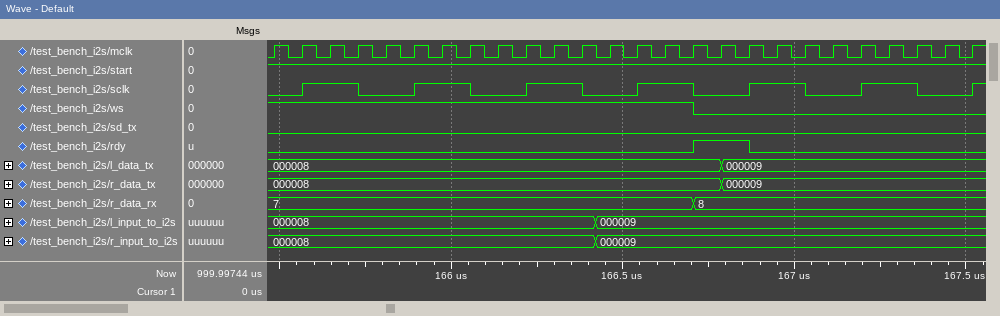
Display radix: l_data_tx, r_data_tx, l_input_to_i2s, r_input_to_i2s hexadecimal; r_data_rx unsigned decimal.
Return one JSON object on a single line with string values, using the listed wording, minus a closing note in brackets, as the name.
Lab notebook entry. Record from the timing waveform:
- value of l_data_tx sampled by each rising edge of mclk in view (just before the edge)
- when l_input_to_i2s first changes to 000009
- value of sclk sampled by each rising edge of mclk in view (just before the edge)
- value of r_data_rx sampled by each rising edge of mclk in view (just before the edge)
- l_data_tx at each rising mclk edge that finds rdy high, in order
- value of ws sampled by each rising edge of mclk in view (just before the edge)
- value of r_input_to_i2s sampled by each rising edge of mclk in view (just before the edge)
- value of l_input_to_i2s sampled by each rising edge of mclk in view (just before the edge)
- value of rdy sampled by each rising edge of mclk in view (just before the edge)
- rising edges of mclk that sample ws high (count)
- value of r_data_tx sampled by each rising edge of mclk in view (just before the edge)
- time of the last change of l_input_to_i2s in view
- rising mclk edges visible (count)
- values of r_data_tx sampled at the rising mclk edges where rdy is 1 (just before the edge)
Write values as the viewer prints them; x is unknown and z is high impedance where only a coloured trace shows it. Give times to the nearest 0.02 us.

{"value of l_data_tx sampled by each rising edge of mclk in view": "000008, 000008, 000008, 000008, 000008, 000008, 000008, 000008, 000008, 000008, 000008, 000008, 000008, 000008, 000008, 000008, 000008, 000009, 000009, 000009, 000009, 000009, 000009, 000009, 000009, 000009", "when l_input_to_i2s first changes to 000009": "166.42 us", "value of sclk sampled by each rising edge of mclk in view": "0 0 1 1 0 0 1 1 0 0 1 1 0 0 1 1 0 0 1 1 0 0 1 1 0 0", "value of r_data_rx sampled by each rising edge of mclk in view": "7, 7, 7, 7, 7, 7, 7, 7, 7, 7, 7, 7, 7, 7, 7, 7, 8, 8, 8, 8, 8, 8, 8, 8, 8, 8", "l_data_tx at each rising mclk edge that finds rdy high, in order": "000008, 000009", "value of ws sampled by each rising edge of mclk in view": "1 1 1 1 1 1 1 1 1 1 1 1 1 1 1 1 0 0 0 0 0 0 0 0 0 0", "value of r_input_to_i2s sampled by each rising edge of mclk in view": "000008, 000008, 000008, 000008, 000008, 000008, 000008, 000008, 000008, 000008, 000008, 000008, 000009, 000009, 000009, 000009, 000009, 000009, 000009, 000009, 000009, 000009, 000009, 000009, 000009, 000009", "value of l_input_to_i2s sampled by each rising edge of mclk in view": "000008, 000008, 000008, 000008, 000008, 000008, 000008, 000008, 000008, 000008, 000008, 000008, 000009, 000009, 000009, 000009, 000009, 000009, 000009, 000009, 000009, 000009, 000009, 000009, 000009, 000009", "value of rdy sampled by each rising edge of mclk in view": "0 0 0 0 0 0 0 0 0 0 0 0 0 0 0 0 1 1 0 0 0 0 0 0 0 0", "rising edges of mclk that sample ws high": "16", "value of r_data_tx sampled by each rising edge of mclk in view": "000008, 000008, 000008, 000008, 000008, 000008, 000008, 000008, 000008, 000008, 000008, 000008, 000008, 000008, 000008, 000008, 000008, 000009, 000009, 000009, 000009, 000009, 000009, 000009, 000009, 000009", "time of the last change of l_input_to_i2s in view": "166.42 us", "rising mclk edges visible": "26", "values of r_data_tx sampled at the rising mclk edges where rdy is 1": "000008, 000009"}
